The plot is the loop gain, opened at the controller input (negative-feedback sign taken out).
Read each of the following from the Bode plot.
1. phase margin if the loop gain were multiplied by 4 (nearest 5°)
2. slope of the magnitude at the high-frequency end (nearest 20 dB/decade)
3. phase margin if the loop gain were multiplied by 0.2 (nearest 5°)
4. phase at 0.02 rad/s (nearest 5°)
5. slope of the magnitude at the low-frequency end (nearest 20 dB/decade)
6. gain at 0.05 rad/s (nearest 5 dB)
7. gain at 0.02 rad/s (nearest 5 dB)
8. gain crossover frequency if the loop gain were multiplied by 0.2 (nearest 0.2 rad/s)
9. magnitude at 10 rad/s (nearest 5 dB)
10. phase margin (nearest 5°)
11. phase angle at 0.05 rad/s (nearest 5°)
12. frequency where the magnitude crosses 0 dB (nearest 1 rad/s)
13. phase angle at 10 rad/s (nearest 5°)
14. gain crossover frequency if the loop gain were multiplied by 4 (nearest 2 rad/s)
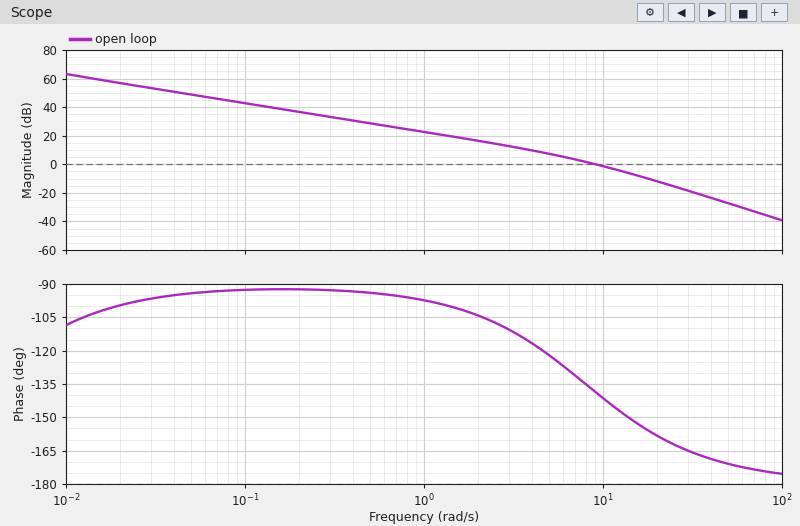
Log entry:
20°
-40 dB/decade
70°
-100°
-20 dB/decade
50 dB
55 dB
2.6 rad/s
0 dB
40°
-95°
9 rad/s
-140°
20 rad/s
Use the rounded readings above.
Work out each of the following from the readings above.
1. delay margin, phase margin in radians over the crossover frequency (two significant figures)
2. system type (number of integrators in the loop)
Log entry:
0.078 s
1
